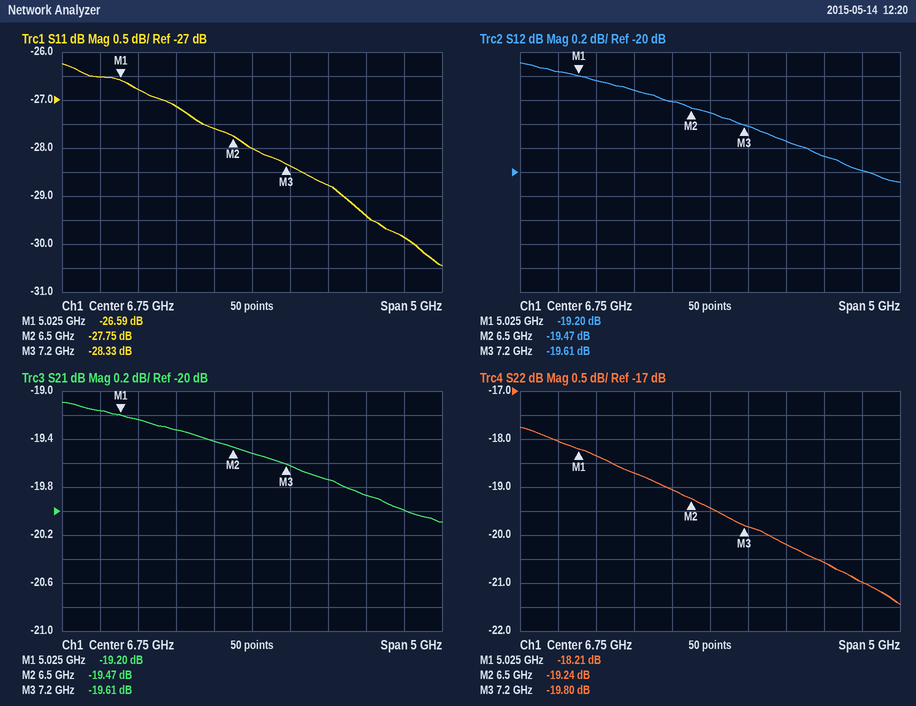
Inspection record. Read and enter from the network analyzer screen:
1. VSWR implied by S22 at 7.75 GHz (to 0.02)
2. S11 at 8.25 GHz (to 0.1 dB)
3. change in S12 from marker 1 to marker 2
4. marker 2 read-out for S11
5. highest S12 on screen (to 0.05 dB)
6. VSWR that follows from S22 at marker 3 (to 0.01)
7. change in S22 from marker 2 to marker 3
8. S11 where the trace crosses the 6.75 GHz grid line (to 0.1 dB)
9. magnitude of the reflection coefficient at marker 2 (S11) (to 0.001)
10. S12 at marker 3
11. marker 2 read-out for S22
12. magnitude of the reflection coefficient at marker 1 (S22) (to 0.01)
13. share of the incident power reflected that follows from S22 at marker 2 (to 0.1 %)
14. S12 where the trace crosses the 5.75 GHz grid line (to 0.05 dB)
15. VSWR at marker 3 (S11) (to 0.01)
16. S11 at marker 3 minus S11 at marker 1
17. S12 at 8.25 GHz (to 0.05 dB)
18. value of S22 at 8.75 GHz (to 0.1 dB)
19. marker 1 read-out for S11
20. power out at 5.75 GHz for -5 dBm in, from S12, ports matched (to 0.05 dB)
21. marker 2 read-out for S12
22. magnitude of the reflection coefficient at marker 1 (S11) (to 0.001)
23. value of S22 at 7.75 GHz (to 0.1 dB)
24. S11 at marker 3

1.22
-29.4 dB
-0.27 dB
-27.75 dB
-19.10 dB
1.23
-0.56 dB
-28.0 dB
0.041
-19.61 dB
-19.24 dB
0.12
1.2 %
-19.30 dB
1.08
-1.74 dB
-19.85 dB
-21.0 dB
-26.59 dB
-24.30 dBm
-19.47 dB
0.047
-20.2 dB
-28.33 dB
